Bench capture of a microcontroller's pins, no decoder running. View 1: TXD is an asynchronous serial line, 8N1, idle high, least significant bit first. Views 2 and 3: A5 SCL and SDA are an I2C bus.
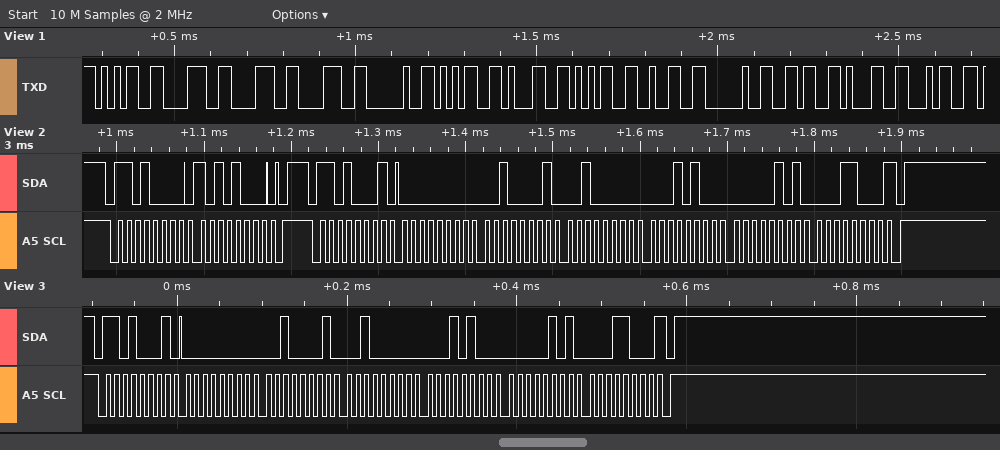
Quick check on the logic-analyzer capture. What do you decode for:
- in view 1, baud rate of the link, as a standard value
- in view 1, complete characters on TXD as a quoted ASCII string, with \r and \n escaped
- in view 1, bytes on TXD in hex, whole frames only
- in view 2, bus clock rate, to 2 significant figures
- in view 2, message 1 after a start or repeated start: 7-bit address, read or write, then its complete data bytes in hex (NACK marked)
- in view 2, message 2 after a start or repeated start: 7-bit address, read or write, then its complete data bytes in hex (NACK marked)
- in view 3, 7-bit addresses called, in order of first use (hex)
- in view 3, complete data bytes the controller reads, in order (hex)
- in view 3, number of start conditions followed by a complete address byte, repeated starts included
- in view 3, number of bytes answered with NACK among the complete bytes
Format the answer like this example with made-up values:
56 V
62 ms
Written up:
57600 baud
"5888 5152 614"
35 38 38 38 20 35 31 35 32 20 36 31 34
100 kHz
0x68 write: A8
0x68 read: 00 21 20 14 05 18 NACK
0x68
00 21 20 14 05 18
1
1
